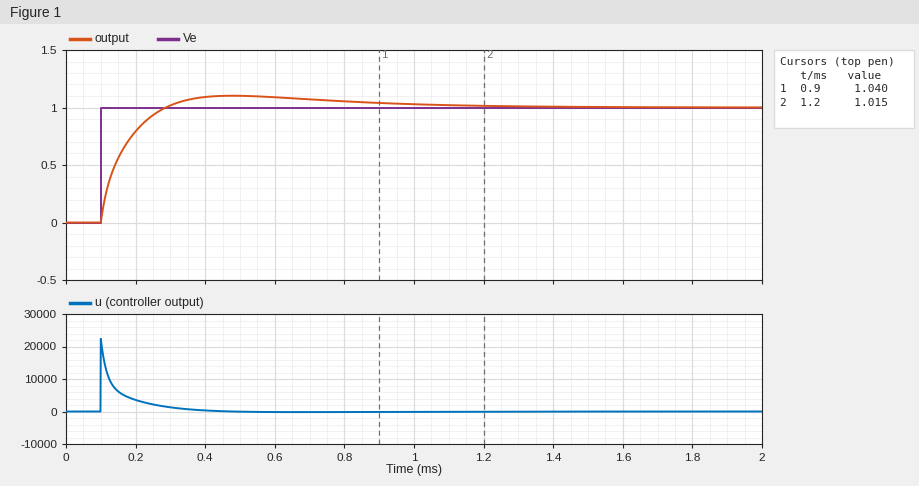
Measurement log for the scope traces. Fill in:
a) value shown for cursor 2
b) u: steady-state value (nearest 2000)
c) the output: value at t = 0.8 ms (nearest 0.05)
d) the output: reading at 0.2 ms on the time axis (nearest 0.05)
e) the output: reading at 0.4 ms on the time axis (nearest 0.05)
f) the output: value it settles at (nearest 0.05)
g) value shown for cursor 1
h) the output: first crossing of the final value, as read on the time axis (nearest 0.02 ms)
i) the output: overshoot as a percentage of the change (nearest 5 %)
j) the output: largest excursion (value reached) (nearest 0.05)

1.015
0
1.05
0.80
1.10
1.00
1.040
0.28 ms
10 %
1.10
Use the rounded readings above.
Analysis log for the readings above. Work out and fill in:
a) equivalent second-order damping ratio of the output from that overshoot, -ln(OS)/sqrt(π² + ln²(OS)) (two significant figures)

0.59
